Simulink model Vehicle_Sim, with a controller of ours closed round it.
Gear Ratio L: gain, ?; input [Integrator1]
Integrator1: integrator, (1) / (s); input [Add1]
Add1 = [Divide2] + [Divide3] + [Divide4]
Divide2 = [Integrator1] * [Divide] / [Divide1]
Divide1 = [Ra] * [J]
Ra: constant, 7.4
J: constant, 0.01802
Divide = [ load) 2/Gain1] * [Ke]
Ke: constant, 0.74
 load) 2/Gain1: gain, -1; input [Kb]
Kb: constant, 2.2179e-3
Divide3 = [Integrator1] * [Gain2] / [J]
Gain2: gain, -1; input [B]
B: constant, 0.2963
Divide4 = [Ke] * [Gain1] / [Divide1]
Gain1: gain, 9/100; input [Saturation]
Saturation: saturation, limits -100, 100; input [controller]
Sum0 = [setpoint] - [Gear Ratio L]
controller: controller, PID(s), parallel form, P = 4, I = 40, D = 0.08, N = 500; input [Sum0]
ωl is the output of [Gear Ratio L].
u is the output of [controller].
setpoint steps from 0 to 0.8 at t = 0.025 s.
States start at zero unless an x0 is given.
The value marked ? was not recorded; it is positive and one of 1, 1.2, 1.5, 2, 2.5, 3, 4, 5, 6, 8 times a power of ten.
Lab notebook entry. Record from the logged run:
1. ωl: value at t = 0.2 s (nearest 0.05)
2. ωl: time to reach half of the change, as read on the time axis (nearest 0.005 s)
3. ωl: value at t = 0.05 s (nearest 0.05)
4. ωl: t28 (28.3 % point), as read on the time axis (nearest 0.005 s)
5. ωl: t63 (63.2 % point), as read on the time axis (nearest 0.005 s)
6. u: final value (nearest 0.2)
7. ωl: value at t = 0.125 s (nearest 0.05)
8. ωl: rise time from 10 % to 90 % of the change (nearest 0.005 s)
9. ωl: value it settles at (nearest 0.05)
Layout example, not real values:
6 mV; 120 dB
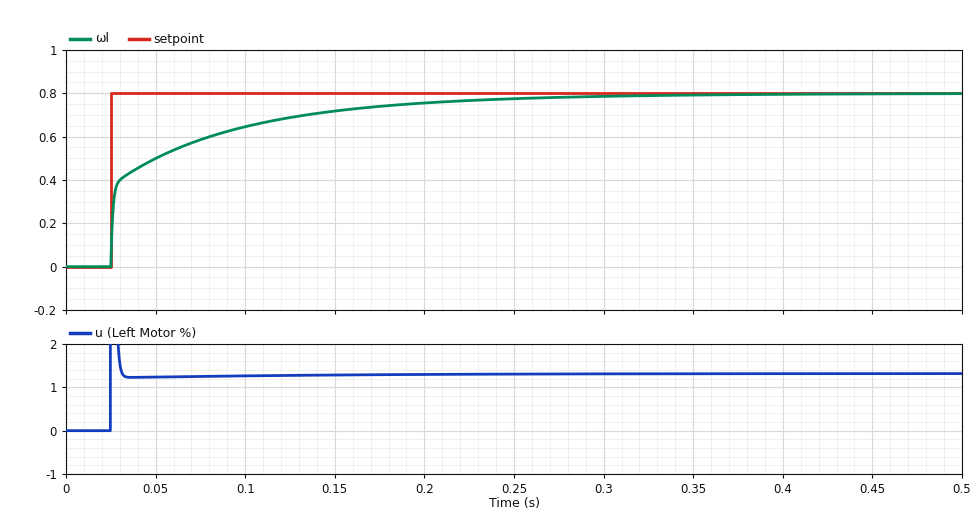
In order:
0.75; 0.030 s; 0.50; 0.025 s; 0.050 s; 1.4; 0.70; 0.125 s; 0.80
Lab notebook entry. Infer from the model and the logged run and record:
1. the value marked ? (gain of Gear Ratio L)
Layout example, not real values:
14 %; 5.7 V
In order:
20
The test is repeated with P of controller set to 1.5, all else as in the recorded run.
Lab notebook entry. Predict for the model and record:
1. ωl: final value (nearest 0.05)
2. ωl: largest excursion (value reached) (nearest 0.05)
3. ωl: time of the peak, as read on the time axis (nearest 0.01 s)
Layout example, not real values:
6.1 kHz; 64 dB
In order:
0.80; 0.85; 0.28 s
